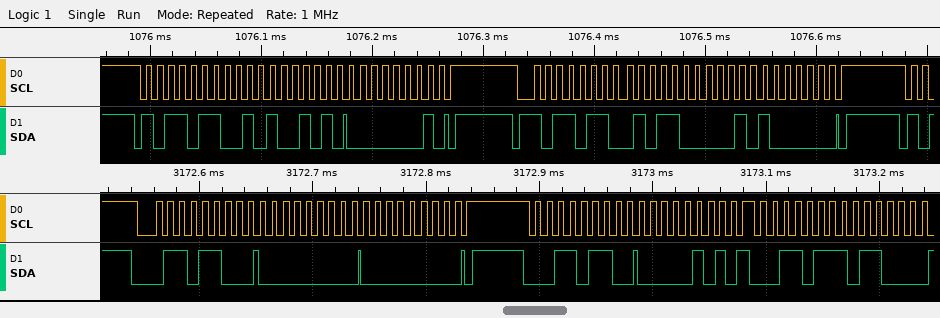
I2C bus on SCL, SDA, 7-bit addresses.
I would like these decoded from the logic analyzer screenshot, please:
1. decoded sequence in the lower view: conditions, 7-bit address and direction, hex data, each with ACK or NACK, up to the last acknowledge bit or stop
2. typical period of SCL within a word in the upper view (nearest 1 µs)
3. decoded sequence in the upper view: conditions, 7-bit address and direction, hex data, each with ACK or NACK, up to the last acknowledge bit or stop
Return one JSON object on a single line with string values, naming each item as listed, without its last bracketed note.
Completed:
{"decoded sequence in the lower view: conditions, 7-bit address and direction, hex data, each with ACK or NACK, up to the last acknowledge bit or stop": "start, address 36 write ACK, 00 ACK, 00 ACK, stop, start, address 1B write ACK, 05 ACK, repeated start, address 1B read ACK", "typical period of SCL within a word in the upper view": "10 µs", "decoded sequence in the upper view: conditions, 7-bit address and direction, hex data, each with ACK or NACK, up to the last acknowledge bit or stop": "start, address 5B write ACK, A5 ACK, 01 ACK, stop, start, address 5B write ACK, B0 ACK, A0 ACK, stop"}
